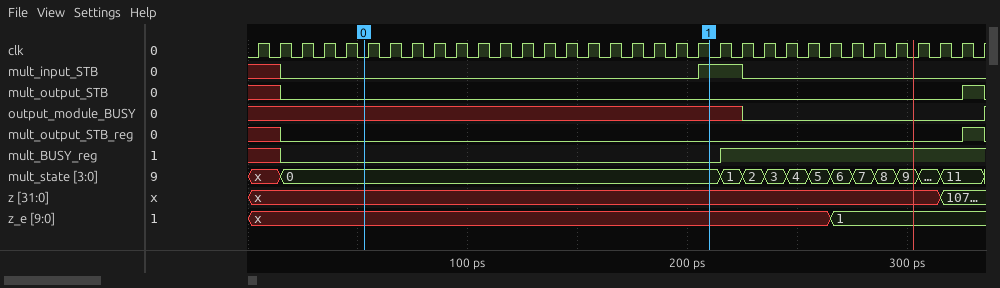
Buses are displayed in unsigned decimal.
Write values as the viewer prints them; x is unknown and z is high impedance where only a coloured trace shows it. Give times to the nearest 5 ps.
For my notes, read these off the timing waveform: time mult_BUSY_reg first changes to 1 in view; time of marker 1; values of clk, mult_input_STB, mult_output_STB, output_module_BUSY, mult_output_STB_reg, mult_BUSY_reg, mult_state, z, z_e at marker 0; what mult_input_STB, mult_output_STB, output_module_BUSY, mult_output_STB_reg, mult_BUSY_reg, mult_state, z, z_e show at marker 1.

215 ps
210 ps
clk=0, mult_input_STB=0, mult_output_STB=0, output_module_BUSY=x, mult_output_STB_reg=0, mult_BUSY_reg=0, mult_state=0, z=x, z_e=x
mult_input_STB=1, mult_output_STB=0, output_module_BUSY=x, mult_output_STB_reg=0, mult_BUSY_reg=0, mult_state=0, z=x, z_e=x
